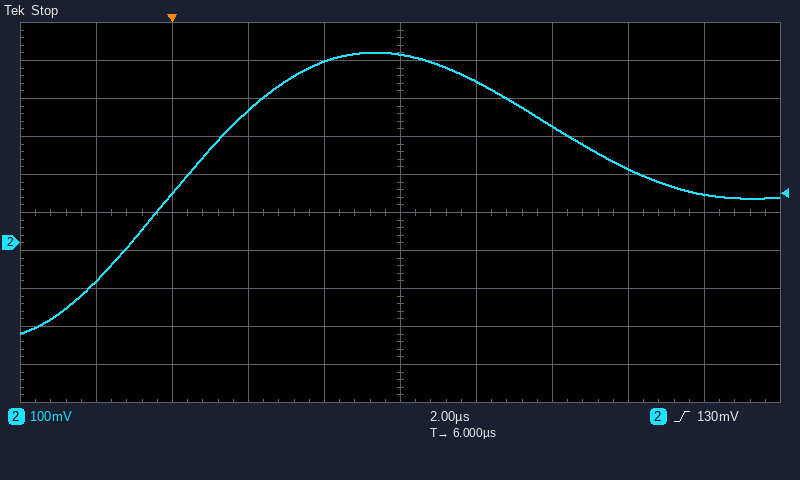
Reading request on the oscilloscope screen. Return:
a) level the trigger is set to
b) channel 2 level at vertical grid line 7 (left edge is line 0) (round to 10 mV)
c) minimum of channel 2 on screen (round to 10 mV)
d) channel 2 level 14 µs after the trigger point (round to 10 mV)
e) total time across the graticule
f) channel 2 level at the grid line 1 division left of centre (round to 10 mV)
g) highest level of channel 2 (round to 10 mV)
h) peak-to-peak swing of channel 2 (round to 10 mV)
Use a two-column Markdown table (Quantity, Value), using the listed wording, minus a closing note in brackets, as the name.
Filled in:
| Quantity | Value |
|---|---|
| level the trigger is set to | 130 mV |
| channel 2 level at vertical grid line 7 (left edge is line 0) | 310 mV |
| minimum of channel 2 on screen | -240 mV |
| channel 2 level 14 µs after the trigger point | 130 mV |
| total time across the graticule | 20 µs |
| channel 2 level at the grid line 1 division left of centre | 480 mV |
| highest level of channel 2 | 500 mV |
| peak-to-peak swing of channel 2 | 740 mV |
